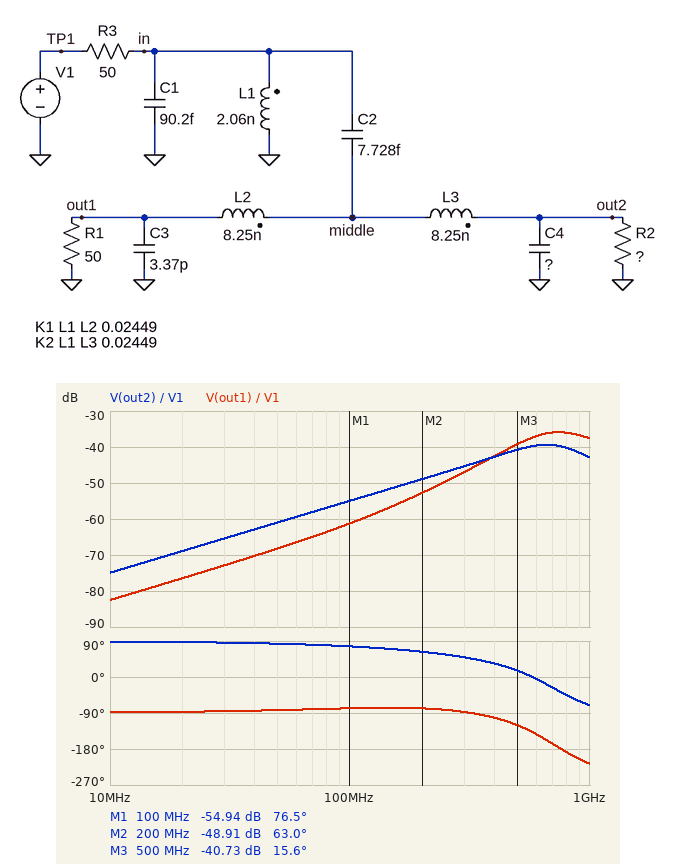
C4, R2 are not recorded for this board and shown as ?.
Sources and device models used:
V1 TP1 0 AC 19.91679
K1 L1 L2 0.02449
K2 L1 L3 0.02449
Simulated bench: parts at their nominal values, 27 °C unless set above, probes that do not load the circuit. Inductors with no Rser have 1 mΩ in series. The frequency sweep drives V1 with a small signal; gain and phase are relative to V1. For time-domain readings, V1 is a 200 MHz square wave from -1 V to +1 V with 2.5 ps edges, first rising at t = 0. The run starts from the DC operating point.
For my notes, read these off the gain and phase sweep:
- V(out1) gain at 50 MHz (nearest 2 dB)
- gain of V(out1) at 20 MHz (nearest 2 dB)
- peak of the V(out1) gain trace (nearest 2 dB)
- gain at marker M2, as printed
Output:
-68 dB
-76 dB
-36 dB
-48.91 dB
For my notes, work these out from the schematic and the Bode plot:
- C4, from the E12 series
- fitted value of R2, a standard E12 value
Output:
8.2 pF
120 Ω
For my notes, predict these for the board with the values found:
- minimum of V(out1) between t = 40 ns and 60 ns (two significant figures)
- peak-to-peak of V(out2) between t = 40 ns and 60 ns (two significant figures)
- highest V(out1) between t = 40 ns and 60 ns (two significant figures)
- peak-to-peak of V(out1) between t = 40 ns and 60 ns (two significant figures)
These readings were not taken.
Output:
-15 mV
23 mV
15 mV
30 mV
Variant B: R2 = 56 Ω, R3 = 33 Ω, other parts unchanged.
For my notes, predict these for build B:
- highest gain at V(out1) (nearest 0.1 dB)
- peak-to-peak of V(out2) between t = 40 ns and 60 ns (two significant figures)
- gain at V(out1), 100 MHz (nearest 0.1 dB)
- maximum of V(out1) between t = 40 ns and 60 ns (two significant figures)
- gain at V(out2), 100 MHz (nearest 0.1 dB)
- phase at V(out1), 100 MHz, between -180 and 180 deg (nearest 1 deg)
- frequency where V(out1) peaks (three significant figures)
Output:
-33.5 dB
28 mV
-54.5 dB
22 mV
-53.8 dB
-93 deg
772 MHz
